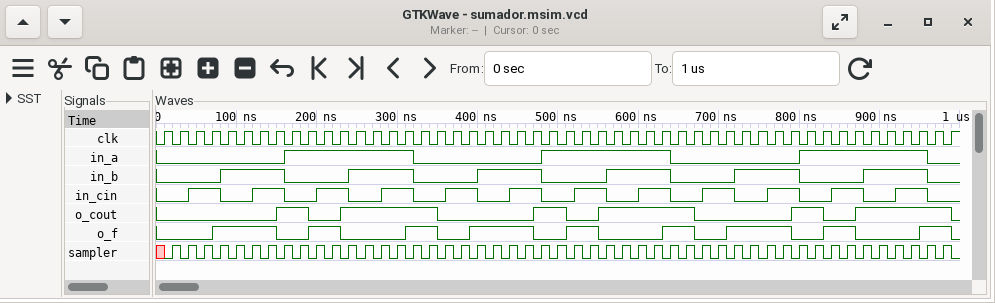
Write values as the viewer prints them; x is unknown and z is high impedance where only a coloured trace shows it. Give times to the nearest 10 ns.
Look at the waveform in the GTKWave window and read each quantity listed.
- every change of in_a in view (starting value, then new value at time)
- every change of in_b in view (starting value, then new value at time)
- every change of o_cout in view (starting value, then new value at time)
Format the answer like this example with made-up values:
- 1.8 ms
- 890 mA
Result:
- 0, 1 at 160 ns, 0 at 320 ns, 1 at 480 ns, 0 at 640 ns, 1 at 800 ns, 0 at 960 ns
- 0, 1 at 80 ns, 0 at 160 ns, 1 at 240 ns, 0 at 320 ns, 1 at 400 ns, 0 at 480 ns, 1 at 560 ns, 0 at 640 ns, 1 at 720 ns, 0 at 800 ns, 1 at 880 ns, 0 at 960 ns
- 0, 1 at 150 ns, 0 at 190 ns, 1 at 230 ns, 0 at 350 ns, 1 at 470 ns, 0 at 510 ns, 1 at 550 ns, 0 at 670 ns, 1 at 790 ns, 0 at 830 ns, 1 at 870 ns, 0 at 990 ns
